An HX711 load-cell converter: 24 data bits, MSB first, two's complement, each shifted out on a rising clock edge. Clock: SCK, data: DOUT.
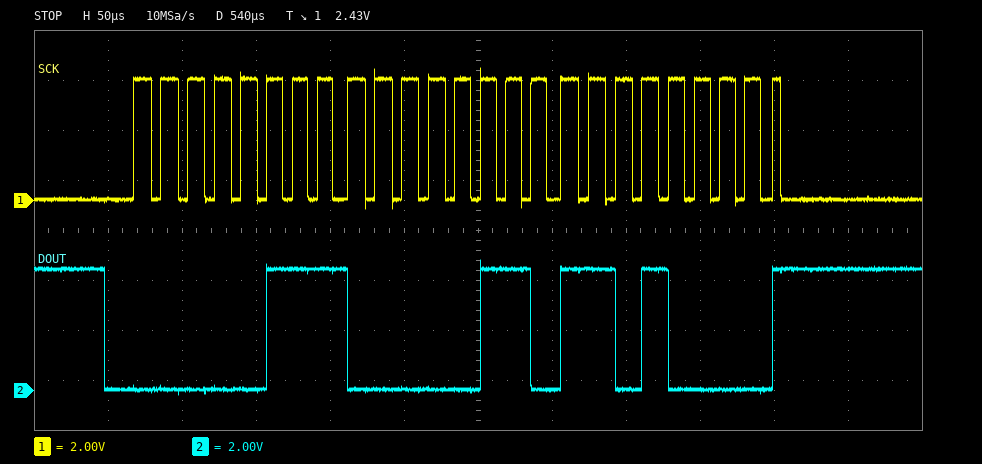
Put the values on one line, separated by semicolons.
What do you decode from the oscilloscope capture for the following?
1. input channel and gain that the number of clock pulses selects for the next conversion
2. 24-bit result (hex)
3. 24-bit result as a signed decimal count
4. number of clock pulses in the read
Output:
channel A, gain 128; 0x0706D0; 460496; 25
